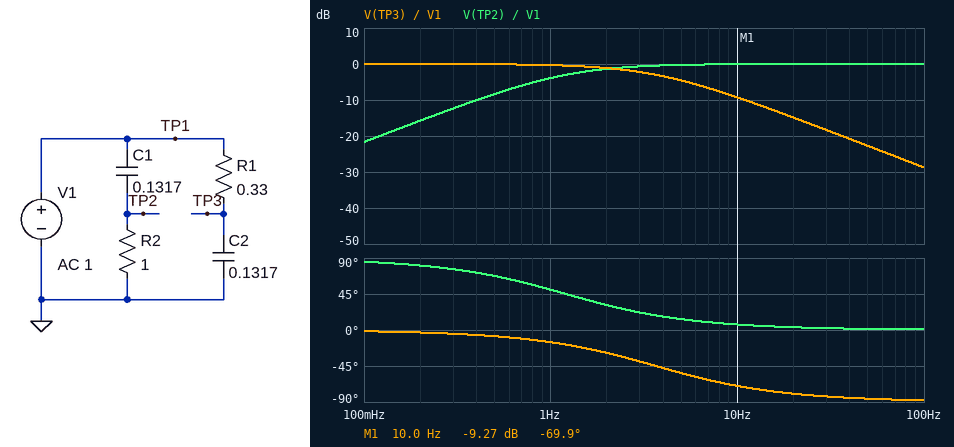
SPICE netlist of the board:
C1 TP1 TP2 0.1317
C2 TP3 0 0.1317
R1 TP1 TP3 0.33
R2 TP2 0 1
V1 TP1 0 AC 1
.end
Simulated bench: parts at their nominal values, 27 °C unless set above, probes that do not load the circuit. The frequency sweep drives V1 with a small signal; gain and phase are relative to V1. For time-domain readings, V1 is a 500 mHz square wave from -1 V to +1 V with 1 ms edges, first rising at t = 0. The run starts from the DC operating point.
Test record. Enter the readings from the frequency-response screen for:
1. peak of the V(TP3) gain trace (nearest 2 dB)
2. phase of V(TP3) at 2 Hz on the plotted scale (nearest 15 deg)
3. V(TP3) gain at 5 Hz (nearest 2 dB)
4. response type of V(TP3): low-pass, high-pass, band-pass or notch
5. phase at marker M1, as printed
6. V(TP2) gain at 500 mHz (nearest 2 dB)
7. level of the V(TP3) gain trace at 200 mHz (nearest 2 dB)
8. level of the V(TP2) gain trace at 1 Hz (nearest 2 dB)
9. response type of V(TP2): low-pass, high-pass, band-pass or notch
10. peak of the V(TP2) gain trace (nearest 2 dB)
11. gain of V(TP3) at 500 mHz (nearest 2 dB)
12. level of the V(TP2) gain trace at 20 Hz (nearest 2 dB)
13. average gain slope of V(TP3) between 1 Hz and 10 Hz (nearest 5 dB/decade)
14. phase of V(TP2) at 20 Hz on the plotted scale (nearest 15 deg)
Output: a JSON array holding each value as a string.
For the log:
["0 dB", "-30 deg", "-4 dB", "low-pass", "-69.9 deg", "-8 dB", "0 dB", "-4 dB", "high-pass", "0 dB", "0 dB", "0 dB", "-10 dB/decade", "0 deg"]
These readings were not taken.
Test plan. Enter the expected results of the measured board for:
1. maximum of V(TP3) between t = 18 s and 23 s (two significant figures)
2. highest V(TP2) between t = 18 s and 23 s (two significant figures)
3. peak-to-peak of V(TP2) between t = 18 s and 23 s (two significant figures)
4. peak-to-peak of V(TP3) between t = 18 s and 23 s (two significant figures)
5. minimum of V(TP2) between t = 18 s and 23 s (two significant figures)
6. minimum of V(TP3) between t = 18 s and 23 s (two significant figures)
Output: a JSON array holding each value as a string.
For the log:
["1.0 V", "2.0 V", "4.0 V", "2.0 V", "-2.0 V", "-1.0 V"]
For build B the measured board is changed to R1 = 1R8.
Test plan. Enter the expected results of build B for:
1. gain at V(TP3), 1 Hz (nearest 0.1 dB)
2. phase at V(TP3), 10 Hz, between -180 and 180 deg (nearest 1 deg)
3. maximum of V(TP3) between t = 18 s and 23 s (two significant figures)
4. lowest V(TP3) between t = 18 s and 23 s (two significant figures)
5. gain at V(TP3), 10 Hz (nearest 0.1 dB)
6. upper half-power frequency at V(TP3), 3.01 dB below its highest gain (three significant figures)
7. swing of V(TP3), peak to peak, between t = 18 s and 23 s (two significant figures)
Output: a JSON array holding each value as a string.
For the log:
["-5.1 dB", "-86 deg", "970 mV", "-970 mV", "-23.5 dB", "671 mHz", "1.9 V"]
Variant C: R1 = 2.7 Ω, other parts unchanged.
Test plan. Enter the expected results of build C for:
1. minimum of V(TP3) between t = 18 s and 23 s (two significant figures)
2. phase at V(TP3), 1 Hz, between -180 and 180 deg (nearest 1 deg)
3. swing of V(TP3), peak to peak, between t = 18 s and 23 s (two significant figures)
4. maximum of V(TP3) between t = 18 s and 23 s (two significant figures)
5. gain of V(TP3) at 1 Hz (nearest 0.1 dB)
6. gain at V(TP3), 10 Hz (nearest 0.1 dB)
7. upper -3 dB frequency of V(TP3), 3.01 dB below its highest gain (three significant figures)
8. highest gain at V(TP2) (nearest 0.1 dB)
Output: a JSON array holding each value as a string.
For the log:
["-890 mV", "-66 deg", "1.8 V", "890 mV", "-7.8 dB", "-27.0 dB", "448 mHz", "0 dB"]
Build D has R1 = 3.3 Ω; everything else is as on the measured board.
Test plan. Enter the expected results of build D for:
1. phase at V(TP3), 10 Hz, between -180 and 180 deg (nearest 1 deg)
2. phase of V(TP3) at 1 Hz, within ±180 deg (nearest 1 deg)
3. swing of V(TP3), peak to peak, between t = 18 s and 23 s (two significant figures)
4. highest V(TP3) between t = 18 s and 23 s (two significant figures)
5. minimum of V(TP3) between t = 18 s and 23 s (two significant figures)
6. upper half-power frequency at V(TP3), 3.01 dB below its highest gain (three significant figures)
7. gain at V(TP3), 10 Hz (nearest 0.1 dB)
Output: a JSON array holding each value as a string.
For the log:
["-88 deg", "-70 deg", "1.6 V", "820 mV", "-820 mV", "366 mHz", "-28.7 dB"]
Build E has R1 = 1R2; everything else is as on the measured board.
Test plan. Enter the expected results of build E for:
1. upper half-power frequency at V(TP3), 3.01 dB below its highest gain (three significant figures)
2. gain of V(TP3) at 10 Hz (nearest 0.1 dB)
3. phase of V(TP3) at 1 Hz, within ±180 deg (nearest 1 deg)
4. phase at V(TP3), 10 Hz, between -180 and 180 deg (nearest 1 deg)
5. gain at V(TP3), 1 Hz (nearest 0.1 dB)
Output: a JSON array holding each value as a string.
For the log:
["1.01 Hz", "-20.0 dB", "-45 deg", "-84 deg", "-3.0 dB"]
